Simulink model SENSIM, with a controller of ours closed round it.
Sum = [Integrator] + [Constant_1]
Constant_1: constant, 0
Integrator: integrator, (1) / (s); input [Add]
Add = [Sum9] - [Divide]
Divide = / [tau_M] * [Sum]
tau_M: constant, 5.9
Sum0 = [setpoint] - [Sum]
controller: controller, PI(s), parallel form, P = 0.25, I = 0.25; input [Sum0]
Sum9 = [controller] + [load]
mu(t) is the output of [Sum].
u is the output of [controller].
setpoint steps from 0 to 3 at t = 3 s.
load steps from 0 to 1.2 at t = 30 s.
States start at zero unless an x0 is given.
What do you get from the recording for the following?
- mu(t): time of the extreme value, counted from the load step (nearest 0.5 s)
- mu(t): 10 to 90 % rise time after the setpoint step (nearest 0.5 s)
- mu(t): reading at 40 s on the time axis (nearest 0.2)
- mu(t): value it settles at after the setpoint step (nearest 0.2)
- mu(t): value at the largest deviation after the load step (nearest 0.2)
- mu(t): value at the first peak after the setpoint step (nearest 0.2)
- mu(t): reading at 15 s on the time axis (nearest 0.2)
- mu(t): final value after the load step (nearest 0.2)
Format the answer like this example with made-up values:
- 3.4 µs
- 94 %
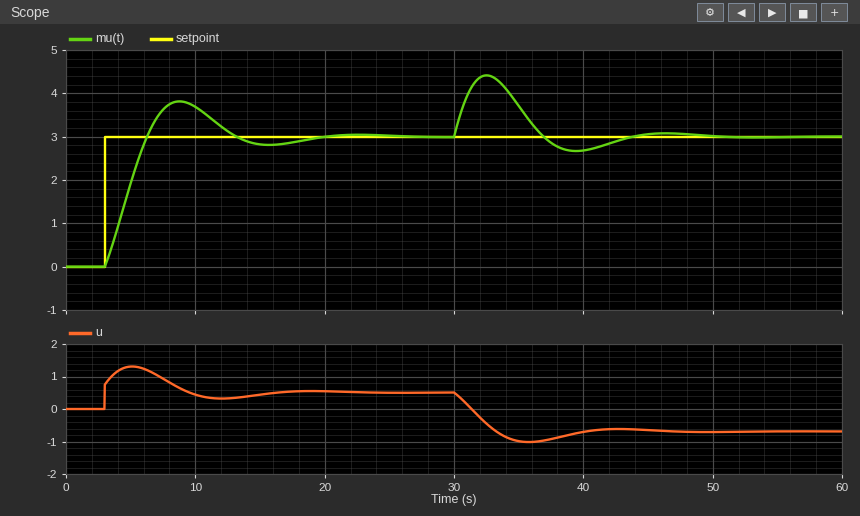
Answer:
- 2.5 s
- 2.5 s
- 2.6
- 3.0
- 4.4
- 3.8
- 2.8
- 3.0
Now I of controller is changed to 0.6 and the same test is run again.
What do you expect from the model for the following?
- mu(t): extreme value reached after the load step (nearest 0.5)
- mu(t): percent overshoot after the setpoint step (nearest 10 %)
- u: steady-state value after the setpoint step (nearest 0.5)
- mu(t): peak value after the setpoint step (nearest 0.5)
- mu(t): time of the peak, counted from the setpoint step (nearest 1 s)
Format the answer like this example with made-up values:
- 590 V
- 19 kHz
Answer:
- 4.0
- 40 %
- 0.5
- 4.5
- 4 s
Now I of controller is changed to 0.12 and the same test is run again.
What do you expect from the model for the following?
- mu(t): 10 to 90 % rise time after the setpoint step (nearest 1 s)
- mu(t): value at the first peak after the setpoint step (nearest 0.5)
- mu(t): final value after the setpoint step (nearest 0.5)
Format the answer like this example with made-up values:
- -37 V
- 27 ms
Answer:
- 4 s
- 3.5
- 3.0
